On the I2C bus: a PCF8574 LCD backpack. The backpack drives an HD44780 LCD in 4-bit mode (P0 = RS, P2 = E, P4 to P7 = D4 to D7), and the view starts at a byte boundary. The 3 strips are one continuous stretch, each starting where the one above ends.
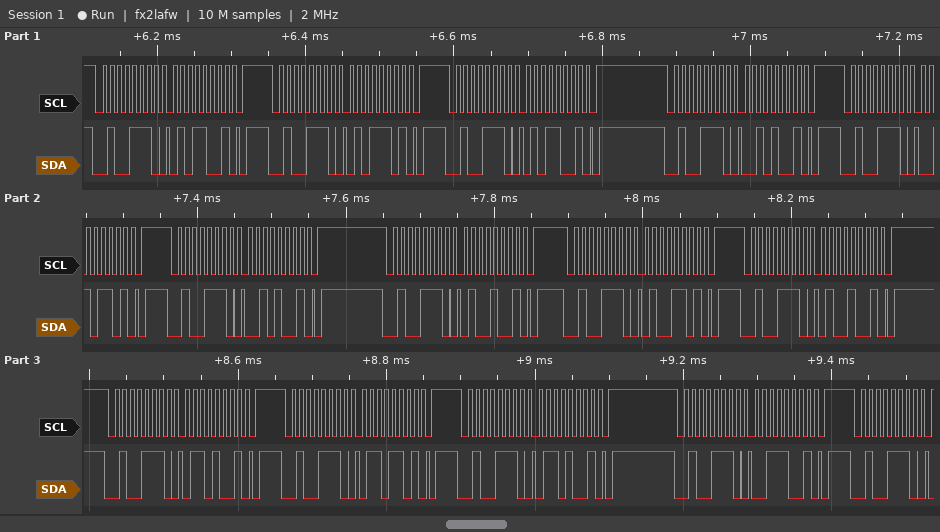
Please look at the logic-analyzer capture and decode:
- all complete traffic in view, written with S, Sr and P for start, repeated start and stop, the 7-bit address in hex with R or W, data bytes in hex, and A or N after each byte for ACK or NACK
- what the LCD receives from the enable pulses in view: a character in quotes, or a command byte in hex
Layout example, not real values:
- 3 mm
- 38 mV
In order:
- S 27W A 59 A P S 27W A 5D A P S 27W A 59 A P S 27W A 29 A P S 27W A 2D A P S 27W A 29 A P S 27W A 49 A P S 27W A 4D A P S 27W A 49 A P S 27W A 69 A P S 27W A 6D A P S 27W A 69 A P S 27W A 39 A P S 27W A
- 'R' 'F'
